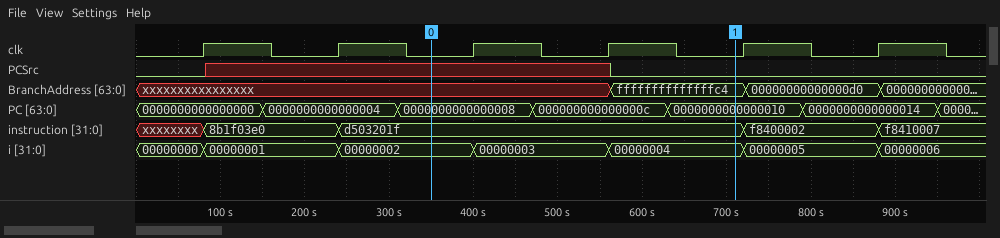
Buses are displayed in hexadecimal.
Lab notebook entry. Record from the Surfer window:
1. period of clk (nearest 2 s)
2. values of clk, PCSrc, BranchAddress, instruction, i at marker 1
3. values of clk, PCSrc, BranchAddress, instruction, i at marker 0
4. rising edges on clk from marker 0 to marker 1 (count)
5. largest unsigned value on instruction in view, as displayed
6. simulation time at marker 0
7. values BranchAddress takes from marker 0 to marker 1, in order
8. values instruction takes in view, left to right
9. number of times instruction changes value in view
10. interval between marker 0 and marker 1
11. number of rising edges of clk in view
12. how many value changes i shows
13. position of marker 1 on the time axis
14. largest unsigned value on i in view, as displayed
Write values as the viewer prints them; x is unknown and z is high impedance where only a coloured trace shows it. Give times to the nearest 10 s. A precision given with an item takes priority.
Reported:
160 s
clk=0, PCSrc=0, BranchAddress=ffffffffffffffc4, instruction=d503201f, i=00000004
clk=0, PCSrc=x, BranchAddress=xxxxxxxxxxxxxxxx, instruction=d503201f, i=00000002
2
f8410007
350 s
xxxxxxxxxxxxxxxx, ffffffffffffffc4
xxxxxxxx, 8b1f03e0, d503201f, f8400002, f8410007
4
360 s
6
6
710 s
00000006
